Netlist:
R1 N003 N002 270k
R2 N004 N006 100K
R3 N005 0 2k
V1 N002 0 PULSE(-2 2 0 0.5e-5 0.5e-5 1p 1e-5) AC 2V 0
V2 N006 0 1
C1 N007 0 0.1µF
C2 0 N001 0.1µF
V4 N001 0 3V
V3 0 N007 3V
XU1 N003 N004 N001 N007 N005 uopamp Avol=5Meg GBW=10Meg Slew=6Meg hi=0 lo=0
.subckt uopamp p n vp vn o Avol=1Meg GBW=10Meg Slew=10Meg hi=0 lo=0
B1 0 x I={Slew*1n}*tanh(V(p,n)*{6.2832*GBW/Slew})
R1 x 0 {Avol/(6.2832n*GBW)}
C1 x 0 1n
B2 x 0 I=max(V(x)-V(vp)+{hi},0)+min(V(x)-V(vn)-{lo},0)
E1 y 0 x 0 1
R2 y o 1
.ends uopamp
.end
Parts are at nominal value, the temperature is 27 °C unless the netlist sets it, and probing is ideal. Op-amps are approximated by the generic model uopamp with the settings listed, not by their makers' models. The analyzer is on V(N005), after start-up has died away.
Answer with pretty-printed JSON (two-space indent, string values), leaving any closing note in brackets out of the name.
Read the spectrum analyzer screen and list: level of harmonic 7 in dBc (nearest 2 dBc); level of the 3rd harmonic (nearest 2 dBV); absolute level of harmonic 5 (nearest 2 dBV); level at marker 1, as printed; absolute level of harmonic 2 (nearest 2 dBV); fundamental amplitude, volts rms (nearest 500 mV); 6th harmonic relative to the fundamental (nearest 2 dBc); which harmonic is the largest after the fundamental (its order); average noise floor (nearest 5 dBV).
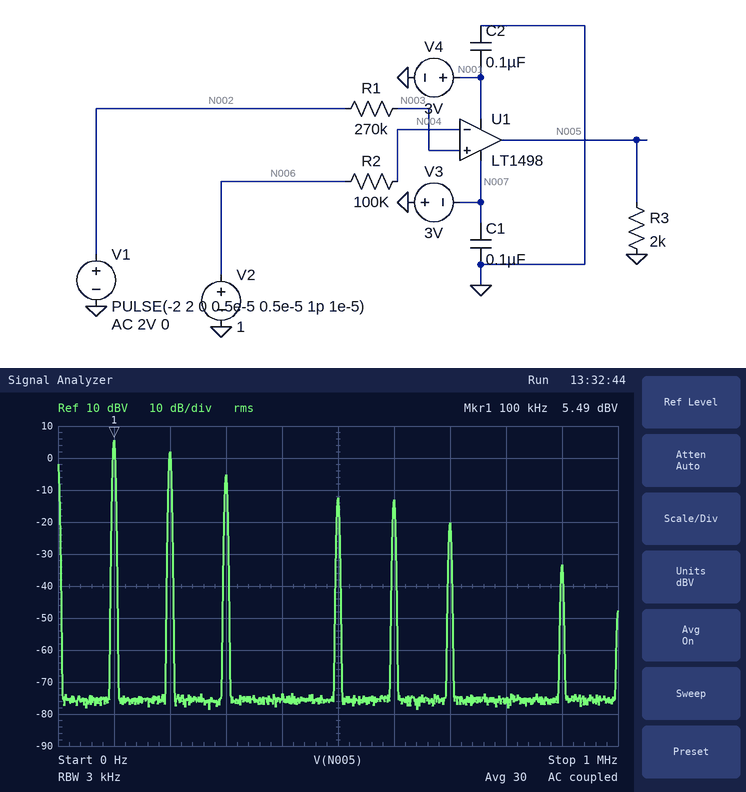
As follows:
{
  "level of harmonic 7 in dBc": "-26 dBc",
  "level of the 3rd harmonic": "-6 dBV",
  "absolute level of harmonic 5": "-12 dBV",
  "level at marker 1, as printed": "5.49 dBV",
  "absolute level of harmonic 2": "2 dBV",
  "fundamental amplitude, volts rms": "2.0 V",
  "6th harmonic relative to the fundamental": "-18 dBc",
  "which harmonic is the largest after the fundamental": "2",
  "average noise floor": "-75 dBV"
}
